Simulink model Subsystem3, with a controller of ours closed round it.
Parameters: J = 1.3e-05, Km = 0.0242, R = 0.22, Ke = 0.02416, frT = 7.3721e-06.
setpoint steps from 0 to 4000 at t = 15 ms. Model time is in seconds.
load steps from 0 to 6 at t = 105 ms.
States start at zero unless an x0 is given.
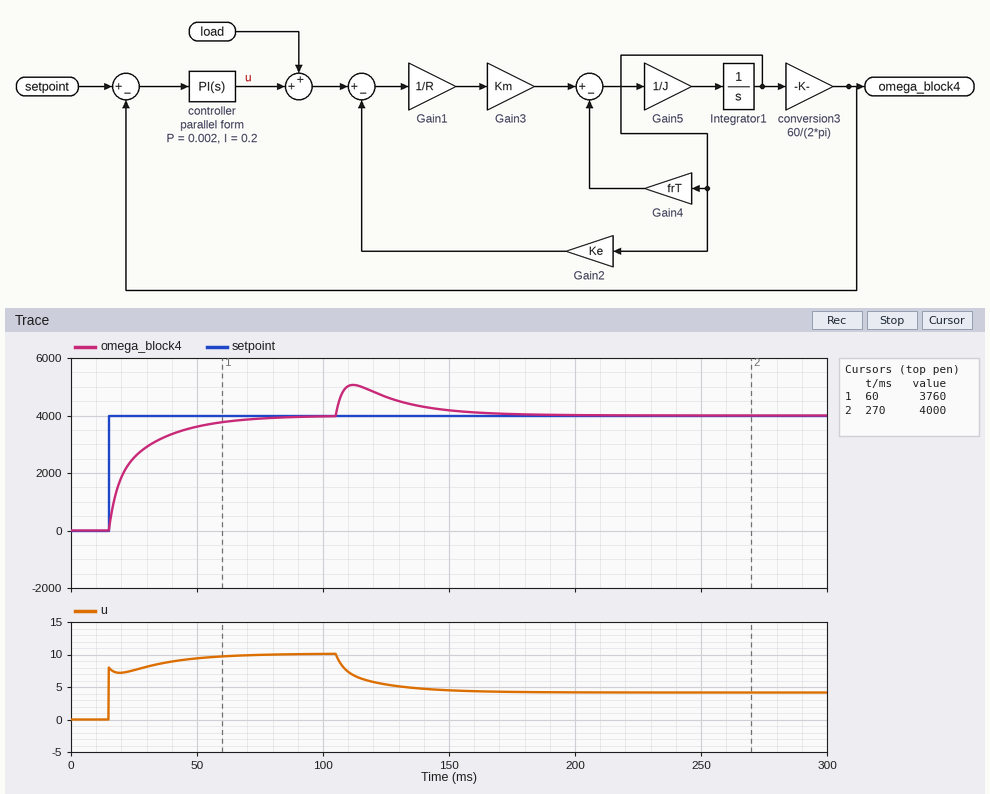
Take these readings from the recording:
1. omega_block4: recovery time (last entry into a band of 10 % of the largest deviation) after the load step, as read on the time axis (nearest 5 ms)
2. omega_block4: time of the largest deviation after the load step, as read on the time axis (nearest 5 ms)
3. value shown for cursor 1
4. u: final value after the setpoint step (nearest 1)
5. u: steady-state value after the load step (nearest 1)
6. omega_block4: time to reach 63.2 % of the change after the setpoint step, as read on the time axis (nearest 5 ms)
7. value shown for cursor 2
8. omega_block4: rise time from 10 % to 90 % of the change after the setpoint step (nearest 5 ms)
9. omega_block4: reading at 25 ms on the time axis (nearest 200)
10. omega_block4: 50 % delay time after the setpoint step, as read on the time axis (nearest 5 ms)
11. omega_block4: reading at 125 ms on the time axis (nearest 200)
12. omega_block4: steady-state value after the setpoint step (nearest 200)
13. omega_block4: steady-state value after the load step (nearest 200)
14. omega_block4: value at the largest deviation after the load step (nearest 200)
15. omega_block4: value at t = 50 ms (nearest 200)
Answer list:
160 ms
110 ms
3760
10
4
25 ms
4000
35 ms
2600
20 ms
4600
4000
4000
5000
3600
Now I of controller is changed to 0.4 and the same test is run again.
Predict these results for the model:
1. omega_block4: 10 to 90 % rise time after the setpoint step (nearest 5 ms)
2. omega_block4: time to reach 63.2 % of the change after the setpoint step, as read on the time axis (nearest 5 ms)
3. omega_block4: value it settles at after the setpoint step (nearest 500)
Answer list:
15 ms
20 ms
4000
